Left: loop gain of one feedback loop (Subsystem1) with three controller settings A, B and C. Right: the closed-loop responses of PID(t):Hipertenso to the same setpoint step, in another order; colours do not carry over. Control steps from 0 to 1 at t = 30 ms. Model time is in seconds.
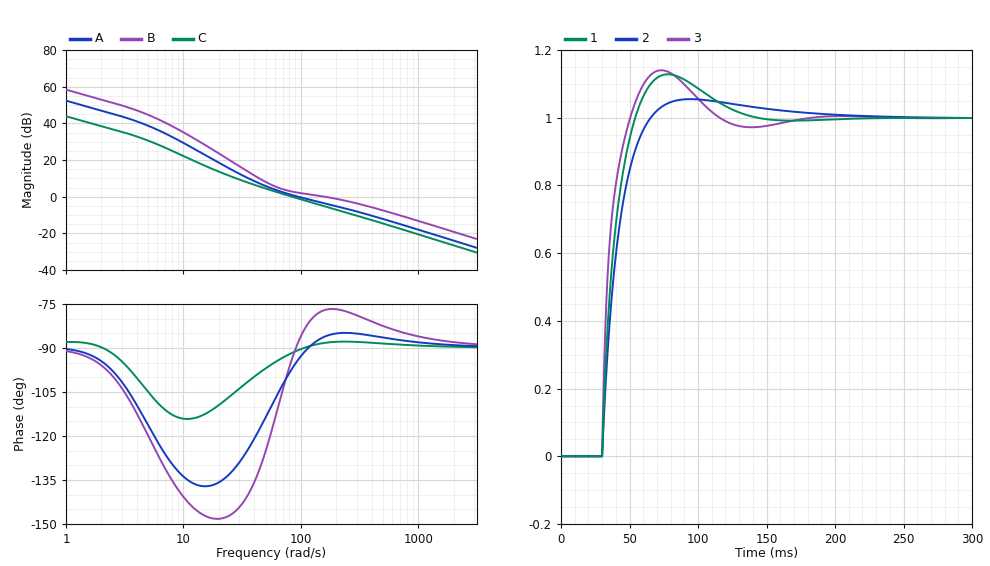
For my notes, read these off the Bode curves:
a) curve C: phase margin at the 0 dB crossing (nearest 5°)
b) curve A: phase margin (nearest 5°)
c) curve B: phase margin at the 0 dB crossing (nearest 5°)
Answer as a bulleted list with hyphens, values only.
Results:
- 90°
- 85°
- 105°
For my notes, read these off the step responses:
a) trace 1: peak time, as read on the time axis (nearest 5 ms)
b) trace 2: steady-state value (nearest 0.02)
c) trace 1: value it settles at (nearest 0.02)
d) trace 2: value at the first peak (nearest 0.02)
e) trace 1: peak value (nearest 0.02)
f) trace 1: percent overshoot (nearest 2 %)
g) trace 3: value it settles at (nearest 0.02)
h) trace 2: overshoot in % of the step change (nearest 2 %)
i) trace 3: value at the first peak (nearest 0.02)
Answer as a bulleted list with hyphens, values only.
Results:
- 80 ms
- 1.00
- 1.00
- 1.06
- 1.12
- 12 %
- 1.00
- 6 %
- 1.14
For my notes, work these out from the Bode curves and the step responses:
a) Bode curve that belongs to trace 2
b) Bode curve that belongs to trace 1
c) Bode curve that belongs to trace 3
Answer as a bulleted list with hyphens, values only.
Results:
- C
- A
- B
